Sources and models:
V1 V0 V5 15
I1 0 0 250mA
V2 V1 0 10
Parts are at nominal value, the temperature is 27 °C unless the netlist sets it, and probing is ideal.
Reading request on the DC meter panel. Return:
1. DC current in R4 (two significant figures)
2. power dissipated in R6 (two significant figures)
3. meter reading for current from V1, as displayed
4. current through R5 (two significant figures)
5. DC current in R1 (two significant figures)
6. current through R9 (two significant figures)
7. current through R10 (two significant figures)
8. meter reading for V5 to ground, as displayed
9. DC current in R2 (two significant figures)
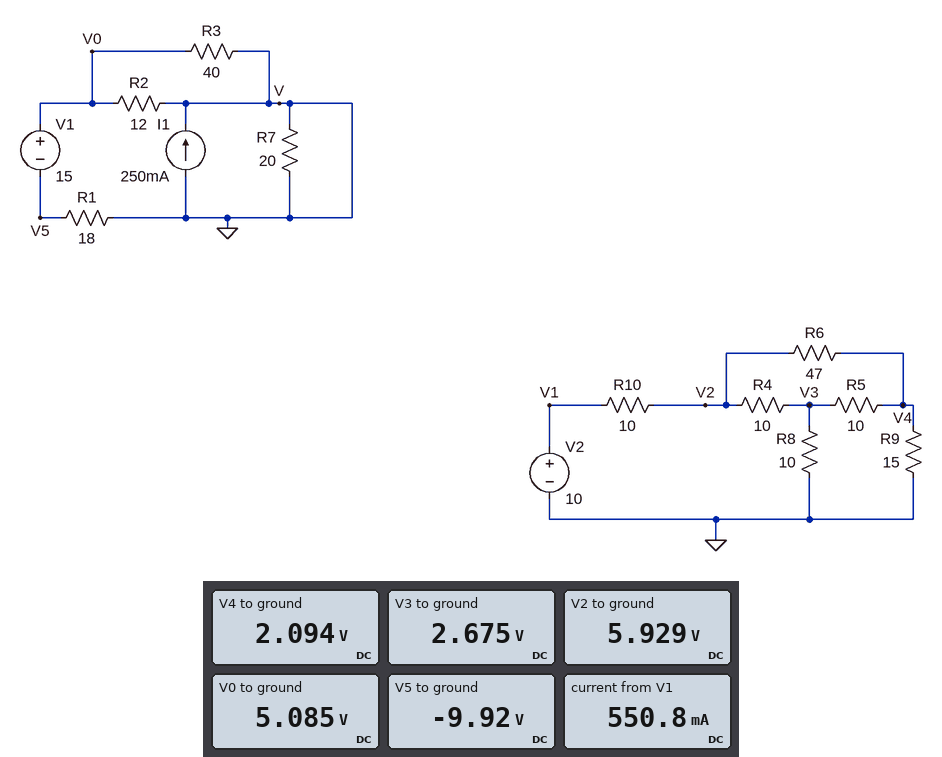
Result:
330 mA
310 mW
550.8 mA
58 mA
550 mA
140 mA
410 mA
-9.92 V
420 mA
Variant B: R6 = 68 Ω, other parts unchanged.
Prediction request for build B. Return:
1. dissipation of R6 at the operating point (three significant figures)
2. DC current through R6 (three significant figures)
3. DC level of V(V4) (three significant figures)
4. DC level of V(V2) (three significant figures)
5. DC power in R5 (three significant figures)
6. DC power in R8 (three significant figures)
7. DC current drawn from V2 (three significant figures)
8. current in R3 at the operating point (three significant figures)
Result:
244 mW
59.9 mA
1.96 V
6.03 V
49.8 mW
709 mW
397 mA
127 mA
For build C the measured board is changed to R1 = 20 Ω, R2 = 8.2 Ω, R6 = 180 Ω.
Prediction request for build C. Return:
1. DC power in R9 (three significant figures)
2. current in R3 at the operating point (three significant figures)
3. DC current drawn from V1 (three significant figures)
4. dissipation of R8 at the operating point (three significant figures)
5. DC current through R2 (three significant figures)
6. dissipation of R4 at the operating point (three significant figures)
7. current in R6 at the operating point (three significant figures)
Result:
201 mW
95.2 mA
560 mA
699 mW
464 mA
1.26 W
24.8 mA
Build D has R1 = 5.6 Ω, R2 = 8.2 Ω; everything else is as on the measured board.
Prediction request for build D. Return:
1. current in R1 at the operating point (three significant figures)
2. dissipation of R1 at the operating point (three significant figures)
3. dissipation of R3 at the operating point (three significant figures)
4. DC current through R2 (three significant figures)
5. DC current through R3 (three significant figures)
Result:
1.21 A
8.19 W
1.69 W
1.00 A
206 mA
